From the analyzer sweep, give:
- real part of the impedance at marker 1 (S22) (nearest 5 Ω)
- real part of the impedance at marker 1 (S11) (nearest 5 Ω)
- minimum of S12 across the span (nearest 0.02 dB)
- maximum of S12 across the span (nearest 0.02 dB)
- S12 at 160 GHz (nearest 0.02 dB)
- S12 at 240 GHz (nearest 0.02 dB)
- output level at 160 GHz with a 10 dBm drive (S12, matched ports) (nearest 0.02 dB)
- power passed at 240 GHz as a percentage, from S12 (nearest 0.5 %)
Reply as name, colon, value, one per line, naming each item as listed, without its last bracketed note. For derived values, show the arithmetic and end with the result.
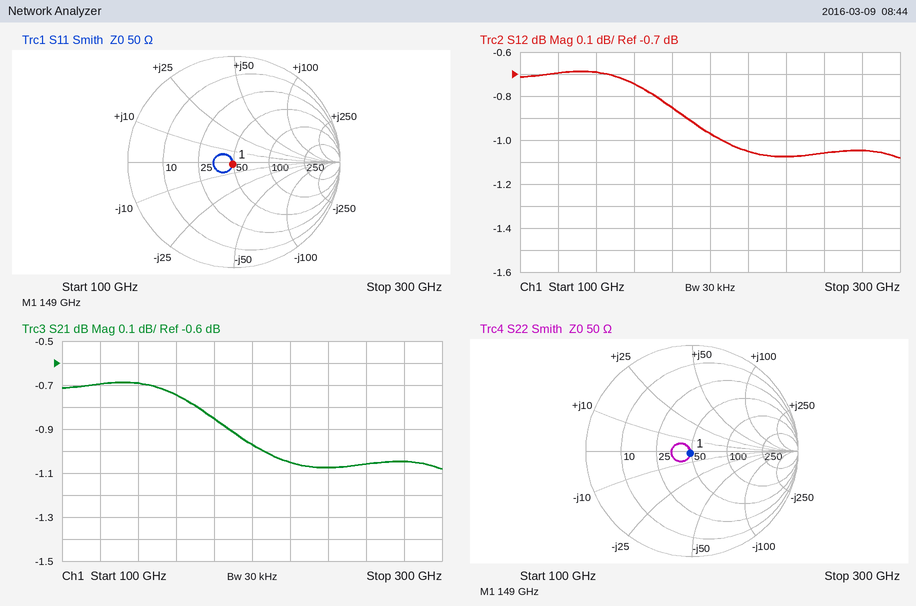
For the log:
real part of the impedance at marker 1 (S22): 50 Ω
real part of the impedance at marker 1 (S11): 50 Ω
minimum of S12 across the span: -1.08 dB
maximum of S12 across the span: -0.68 dB
S12 at 160 GHz: -0.74 dB
S12 at 240 GHz: -1.08 dB
output level at 160 GHz with a 10 dBm drive (S12, matched ports): 10 dBm + (-0.74 dB) = 9.26 dBm
power passed at 240 GHz as a percentage, from S12: 10^(-1.08/10) ≈ 78.0 %
